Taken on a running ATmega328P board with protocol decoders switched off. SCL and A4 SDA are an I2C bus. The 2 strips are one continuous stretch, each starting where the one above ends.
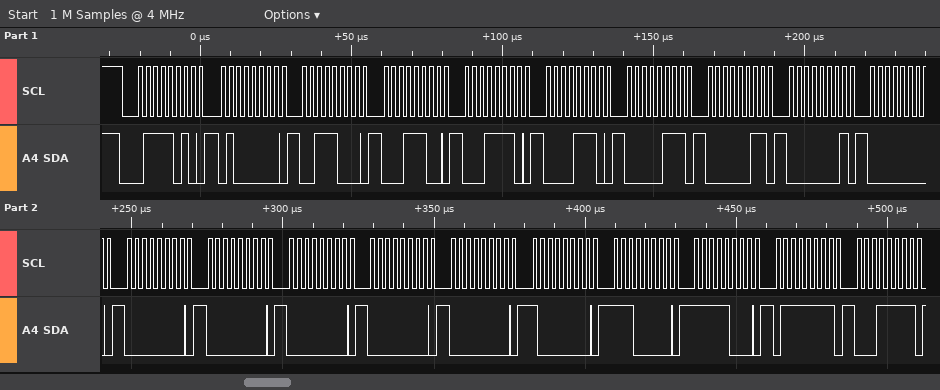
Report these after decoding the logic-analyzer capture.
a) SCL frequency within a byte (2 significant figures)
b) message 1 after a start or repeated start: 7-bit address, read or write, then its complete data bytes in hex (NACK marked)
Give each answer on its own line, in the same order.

400 kHz
0x3D write: 40 38 1C 1E 0E 07 03 01 00 00 00 00 00 00 80 E0 F8 7F 1F
